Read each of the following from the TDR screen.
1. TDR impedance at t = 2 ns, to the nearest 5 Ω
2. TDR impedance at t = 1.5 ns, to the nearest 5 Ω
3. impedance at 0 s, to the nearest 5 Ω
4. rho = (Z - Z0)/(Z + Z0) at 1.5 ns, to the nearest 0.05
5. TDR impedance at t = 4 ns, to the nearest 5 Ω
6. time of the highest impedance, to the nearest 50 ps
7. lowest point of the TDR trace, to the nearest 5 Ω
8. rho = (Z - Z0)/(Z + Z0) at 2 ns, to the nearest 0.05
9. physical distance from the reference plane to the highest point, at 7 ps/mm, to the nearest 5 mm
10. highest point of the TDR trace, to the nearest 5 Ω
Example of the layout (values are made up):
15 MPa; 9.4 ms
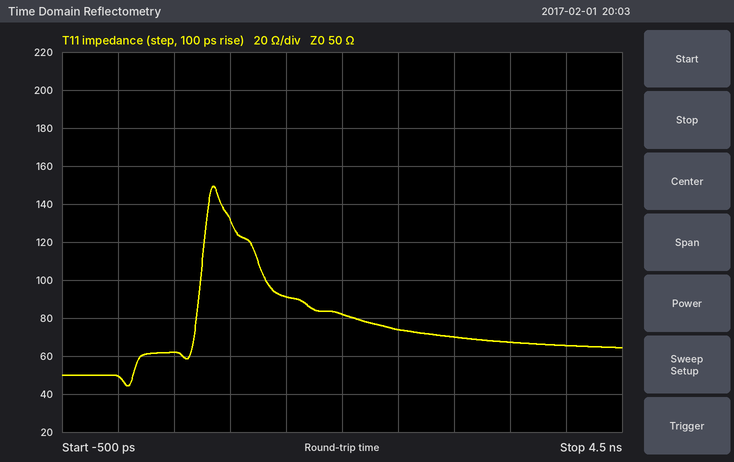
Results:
80 Ω; 90 Ω; 50 Ω; +0.30; 65 Ω; 850 ps; 45 Ω; +0.25; 60 mm; 150 Ω
